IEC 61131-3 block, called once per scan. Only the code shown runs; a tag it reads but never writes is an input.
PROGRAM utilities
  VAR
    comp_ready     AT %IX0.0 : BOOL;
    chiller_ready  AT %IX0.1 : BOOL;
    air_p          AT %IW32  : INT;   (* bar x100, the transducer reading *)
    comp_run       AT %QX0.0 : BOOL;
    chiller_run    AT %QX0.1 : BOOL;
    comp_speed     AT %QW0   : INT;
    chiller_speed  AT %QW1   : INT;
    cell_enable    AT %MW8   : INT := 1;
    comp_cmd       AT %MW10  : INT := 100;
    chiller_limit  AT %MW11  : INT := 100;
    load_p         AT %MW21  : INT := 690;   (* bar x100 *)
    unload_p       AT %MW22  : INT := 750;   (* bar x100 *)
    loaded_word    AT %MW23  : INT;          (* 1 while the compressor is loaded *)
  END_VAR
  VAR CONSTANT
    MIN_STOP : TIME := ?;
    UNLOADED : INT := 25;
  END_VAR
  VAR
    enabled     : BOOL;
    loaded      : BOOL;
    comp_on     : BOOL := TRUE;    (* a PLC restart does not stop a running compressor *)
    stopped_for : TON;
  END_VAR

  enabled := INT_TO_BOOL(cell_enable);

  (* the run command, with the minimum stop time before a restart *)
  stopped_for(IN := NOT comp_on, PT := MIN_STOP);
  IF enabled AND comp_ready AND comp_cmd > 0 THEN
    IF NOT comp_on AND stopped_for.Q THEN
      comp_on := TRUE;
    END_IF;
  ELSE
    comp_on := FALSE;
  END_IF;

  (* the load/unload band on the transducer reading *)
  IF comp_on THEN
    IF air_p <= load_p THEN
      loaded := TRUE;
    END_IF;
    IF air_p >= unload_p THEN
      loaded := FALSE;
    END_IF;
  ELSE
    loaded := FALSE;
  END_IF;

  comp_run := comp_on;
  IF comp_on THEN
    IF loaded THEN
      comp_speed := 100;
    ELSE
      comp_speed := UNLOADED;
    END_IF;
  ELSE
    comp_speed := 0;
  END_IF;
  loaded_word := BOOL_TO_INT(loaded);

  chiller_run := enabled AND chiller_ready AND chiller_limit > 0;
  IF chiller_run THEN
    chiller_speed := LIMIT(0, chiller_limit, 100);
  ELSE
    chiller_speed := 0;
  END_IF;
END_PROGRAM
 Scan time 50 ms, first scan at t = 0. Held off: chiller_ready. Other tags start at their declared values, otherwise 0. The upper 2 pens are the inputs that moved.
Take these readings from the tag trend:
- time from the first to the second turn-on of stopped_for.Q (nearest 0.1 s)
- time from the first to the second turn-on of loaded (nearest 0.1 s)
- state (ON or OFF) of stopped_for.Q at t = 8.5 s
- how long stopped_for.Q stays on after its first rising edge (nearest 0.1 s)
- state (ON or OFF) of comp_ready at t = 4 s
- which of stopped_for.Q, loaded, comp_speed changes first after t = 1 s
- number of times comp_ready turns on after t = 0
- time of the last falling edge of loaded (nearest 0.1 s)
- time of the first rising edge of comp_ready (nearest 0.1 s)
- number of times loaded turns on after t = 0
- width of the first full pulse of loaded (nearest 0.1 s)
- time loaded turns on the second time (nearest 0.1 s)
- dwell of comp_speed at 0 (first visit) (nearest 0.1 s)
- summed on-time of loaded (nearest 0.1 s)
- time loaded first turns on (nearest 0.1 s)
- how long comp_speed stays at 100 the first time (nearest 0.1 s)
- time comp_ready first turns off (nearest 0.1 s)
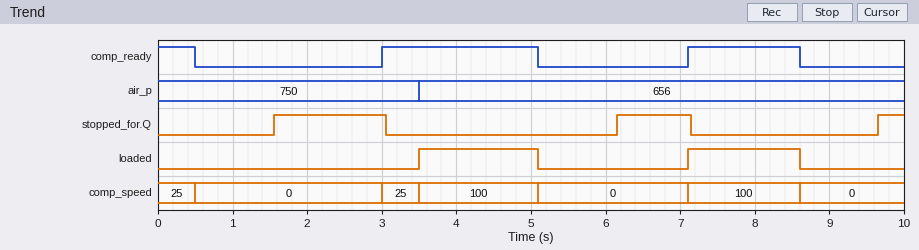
4.6 s
3.6 s
OFF
1.5 s
ON
stopped_for.Q
2
8.6 s
3.0 s
2
1.6 s
7.1 s
2.5 s
3.1 s
3.5 s
1.6 s
0.5 s
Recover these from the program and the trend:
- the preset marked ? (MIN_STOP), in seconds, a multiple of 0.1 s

1.0 s
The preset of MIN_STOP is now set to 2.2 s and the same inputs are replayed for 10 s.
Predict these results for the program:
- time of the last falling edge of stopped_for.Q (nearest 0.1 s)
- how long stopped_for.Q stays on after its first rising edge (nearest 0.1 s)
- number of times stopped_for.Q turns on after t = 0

7.4 s
0.3 s
2
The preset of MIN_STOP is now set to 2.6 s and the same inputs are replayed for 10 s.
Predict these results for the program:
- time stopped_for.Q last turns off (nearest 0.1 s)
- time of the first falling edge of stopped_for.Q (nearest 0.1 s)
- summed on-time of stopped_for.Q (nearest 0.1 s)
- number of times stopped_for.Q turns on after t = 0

7.8 s
3.2 s
0.1 s
2
